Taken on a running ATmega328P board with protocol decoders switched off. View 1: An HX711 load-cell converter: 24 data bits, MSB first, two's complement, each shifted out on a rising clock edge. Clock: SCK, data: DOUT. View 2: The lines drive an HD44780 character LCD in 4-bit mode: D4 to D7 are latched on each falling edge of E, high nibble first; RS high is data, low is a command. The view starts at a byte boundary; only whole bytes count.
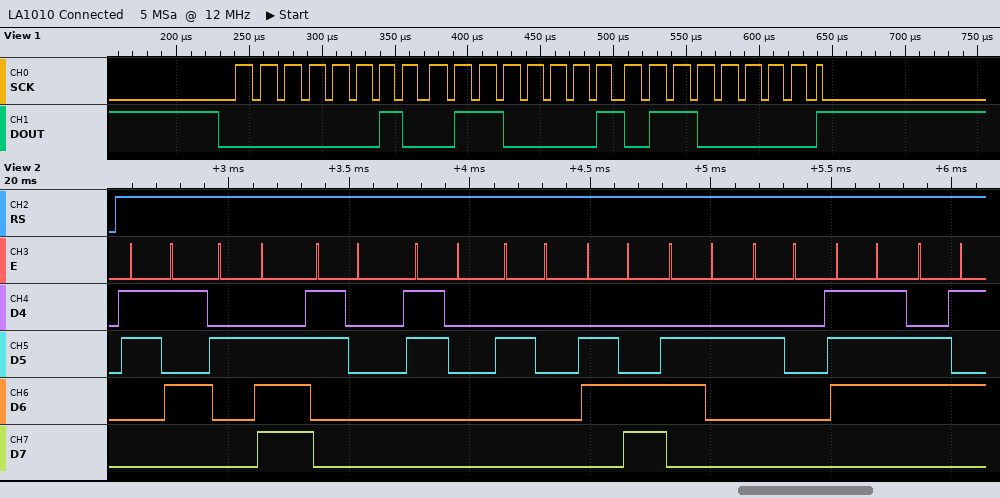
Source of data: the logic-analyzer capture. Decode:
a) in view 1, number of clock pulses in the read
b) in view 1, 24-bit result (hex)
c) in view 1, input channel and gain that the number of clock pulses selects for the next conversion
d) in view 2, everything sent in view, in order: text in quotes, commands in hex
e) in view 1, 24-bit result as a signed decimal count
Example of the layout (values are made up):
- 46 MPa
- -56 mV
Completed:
- 25
- 0x026160
- channel A, gain 128
- "5.00 lb we"
- 156000
